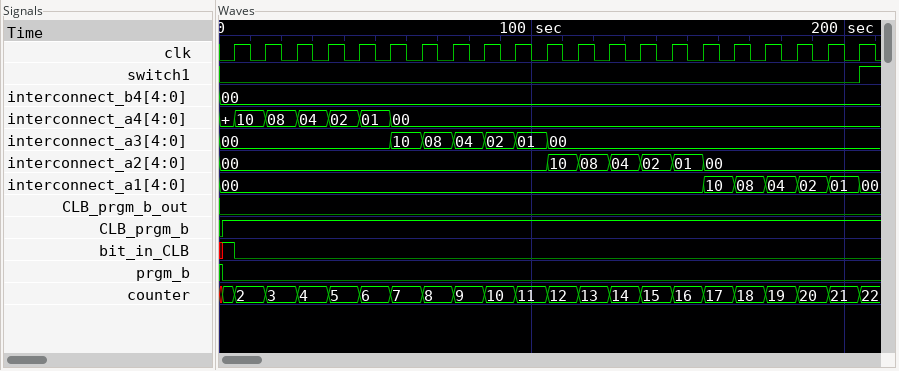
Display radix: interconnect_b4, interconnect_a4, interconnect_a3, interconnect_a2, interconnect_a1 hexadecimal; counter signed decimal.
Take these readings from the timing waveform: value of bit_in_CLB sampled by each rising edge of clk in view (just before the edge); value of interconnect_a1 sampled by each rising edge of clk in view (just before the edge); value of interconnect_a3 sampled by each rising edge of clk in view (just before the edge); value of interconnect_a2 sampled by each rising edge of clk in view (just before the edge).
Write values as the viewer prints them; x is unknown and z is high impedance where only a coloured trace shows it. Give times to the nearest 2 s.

1 0 0 0 0 0 0 0 0 0 0 0 0 0 0 0 0 0 0 0 0
00, 00, 00, 00, 00, 00, 00, 00, 00, 00, 00, 00, 00, 00, 00, 00, 10, 08, 04, 02, 01
00, 00, 00, 00, 00, 00, 10, 08, 04, 02, 01, 00, 00, 00, 00, 00, 00, 00, 00, 00, 00
00, 00, 00, 00, 00, 00, 00, 00, 00, 00, 00, 10, 08, 04, 02, 01, 00, 00, 00, 00, 00
